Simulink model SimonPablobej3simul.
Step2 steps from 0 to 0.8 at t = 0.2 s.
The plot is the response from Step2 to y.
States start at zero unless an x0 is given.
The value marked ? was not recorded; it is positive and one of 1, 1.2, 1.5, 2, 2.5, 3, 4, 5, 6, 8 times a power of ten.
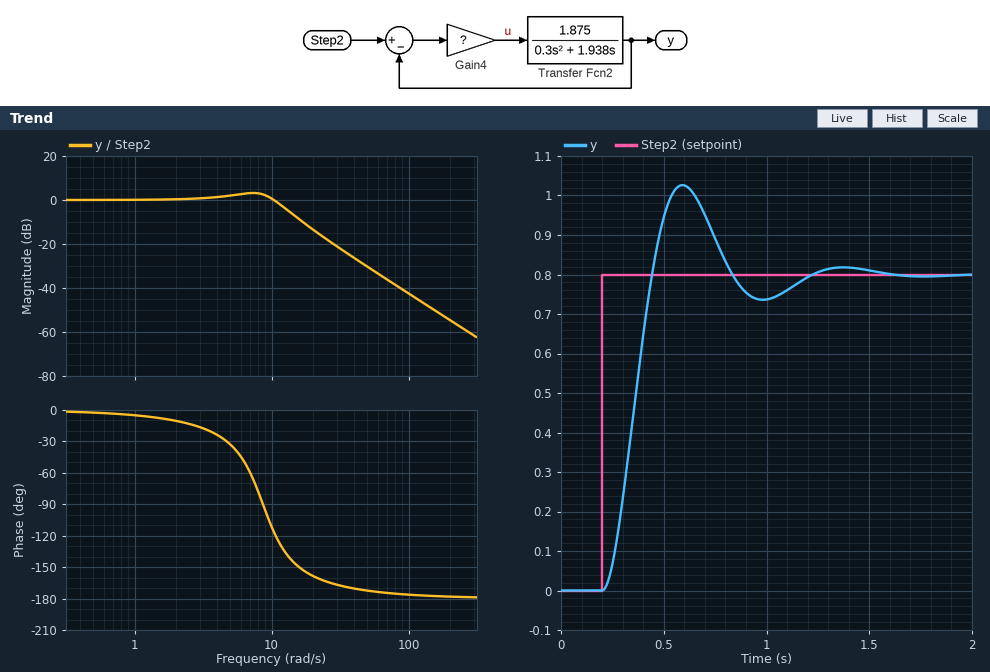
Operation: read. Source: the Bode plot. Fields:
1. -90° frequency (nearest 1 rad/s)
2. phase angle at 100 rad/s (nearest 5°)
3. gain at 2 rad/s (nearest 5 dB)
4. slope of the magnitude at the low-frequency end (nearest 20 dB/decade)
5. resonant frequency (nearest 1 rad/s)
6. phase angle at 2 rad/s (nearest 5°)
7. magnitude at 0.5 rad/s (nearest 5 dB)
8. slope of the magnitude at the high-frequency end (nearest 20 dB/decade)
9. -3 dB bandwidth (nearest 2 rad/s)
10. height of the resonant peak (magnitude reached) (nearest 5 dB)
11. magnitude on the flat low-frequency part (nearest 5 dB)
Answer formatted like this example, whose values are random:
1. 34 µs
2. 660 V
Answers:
1. 9 rad/s
2. -175°
3. 0 dB
4. 0 dB/decade
5. 7 rad/s
6. -10°
7. 0 dB
8. -40 dB/decade
9. 12 rad/s
10. 5 dB
11. 0 dB
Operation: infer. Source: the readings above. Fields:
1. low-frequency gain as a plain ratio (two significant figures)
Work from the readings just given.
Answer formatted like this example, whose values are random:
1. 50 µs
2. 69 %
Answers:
1. 1.0
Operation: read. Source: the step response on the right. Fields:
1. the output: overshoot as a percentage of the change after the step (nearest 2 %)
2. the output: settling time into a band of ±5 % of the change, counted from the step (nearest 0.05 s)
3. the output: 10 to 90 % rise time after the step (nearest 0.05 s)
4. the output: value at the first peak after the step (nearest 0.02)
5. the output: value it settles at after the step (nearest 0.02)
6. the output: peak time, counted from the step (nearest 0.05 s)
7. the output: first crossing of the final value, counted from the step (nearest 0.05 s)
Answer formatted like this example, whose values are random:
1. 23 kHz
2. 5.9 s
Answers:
1. 28 %
2. 0.90 s
3. 0.15 s
4. 1.02
5. 0.80
6. 0.40 s
7. 0.25 s
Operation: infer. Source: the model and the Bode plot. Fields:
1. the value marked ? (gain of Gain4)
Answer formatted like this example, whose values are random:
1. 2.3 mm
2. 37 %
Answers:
1. 12
